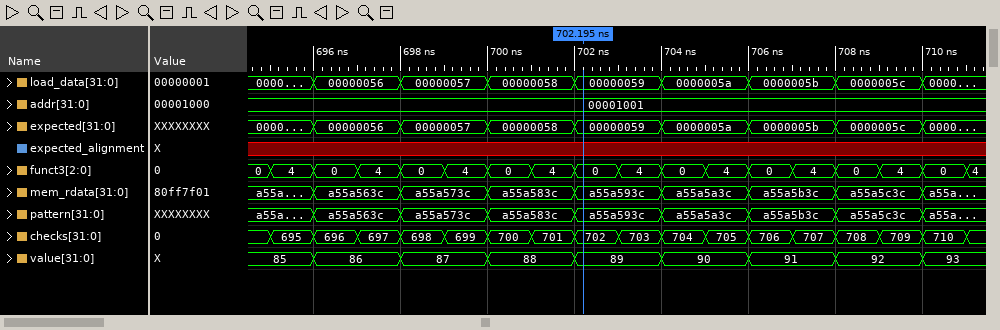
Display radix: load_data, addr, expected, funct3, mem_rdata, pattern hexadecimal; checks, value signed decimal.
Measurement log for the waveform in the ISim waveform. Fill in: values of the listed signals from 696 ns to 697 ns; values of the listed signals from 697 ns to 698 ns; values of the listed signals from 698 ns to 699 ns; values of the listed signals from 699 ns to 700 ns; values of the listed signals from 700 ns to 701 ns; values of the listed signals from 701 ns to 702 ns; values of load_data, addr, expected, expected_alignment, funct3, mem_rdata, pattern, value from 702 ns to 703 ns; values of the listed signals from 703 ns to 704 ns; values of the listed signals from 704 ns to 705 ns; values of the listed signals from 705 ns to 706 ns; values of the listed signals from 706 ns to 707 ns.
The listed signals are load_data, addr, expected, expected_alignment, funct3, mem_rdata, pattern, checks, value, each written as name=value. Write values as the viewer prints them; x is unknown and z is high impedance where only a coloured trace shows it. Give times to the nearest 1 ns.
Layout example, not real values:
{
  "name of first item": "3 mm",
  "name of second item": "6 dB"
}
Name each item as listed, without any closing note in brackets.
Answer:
{
  "values of the listed signals from 696 ns to 697 ns": "load_data=00000056, addr=00001001, expected=00000056, expected_alignment=x, funct3=0, mem_rdata=a55a563c, pattern=a55a563c, checks=696, value=86",
  "values of the listed signals from 697 ns to 698 ns": "load_data=00000056, addr=00001001, expected=00000056, expected_alignment=x, funct3=4, mem_rdata=a55a563c, pattern=a55a563c, checks=697, value=86",
  "values of the listed signals from 698 ns to 699 ns": "load_data=00000057, addr=00001001, expected=00000057, expected_alignment=x, funct3=0, mem_rdata=a55a573c, pattern=a55a573c, checks=698, value=87",
  "values of the listed signals from 699 ns to 700 ns": "load_data=00000057, addr=00001001, expected=00000057, expected_alignment=x, funct3=4, mem_rdata=a55a573c, pattern=a55a573c, checks=699, value=87",
  "values of the listed signals from 700 ns to 701 ns": "load_data=00000058, addr=00001001, expected=00000058, expected_alignment=x, funct3=0, mem_rdata=a55a583c, pattern=a55a583c, checks=700, value=88",
  "values of the listed signals from 701 ns to 702 ns": "load_data=00000058, addr=00001001, expected=00000058, expected_alignment=x, funct3=4, mem_rdata=a55a583c, pattern=a55a583c, checks=701, value=88",
  "values of load_data, addr, expected, expected_alignment, funct3, mem_rdata, pattern, value from 702 ns to 703 ns": "load_data=00000059, addr=00001001, expected=00000059, expected_alignment=x, funct3=0, mem_rdata=a55a593c, pattern=a55a593c, value=89",
  "values of the listed signals from 703 ns to 704 ns": "load_data=00000059, addr=00001001, expected=00000059, expected_alignment=x, funct3=4, mem_rdata=a55a593c, pattern=a55a593c, checks=703, value=89",
  "values of the listed signals from 704 ns to 705 ns": "load_data=0000005a, addr=00001001, expected=0000005a, expected_alignment=x, funct3=0, mem_rdata=a55a5a3c, pattern=a55a5a3c, checks=704, value=90",
  "values of the listed signals from 705 ns to 706 ns": "load_data=0000005a, addr=00001001, expected=0000005a, expected_alignment=x, funct3=4, mem_rdata=a55a5a3c, pattern=a55a5a3c, checks=705, value=90",
  "values of the listed signals from 706 ns to 707 ns": "load_data=0000005b, addr=00001001, expected=0000005b, expected_alignment=x, funct3=0, mem_rdata=a55a5b3c, pattern=a55a5b3c, checks=706, value=91"
}
